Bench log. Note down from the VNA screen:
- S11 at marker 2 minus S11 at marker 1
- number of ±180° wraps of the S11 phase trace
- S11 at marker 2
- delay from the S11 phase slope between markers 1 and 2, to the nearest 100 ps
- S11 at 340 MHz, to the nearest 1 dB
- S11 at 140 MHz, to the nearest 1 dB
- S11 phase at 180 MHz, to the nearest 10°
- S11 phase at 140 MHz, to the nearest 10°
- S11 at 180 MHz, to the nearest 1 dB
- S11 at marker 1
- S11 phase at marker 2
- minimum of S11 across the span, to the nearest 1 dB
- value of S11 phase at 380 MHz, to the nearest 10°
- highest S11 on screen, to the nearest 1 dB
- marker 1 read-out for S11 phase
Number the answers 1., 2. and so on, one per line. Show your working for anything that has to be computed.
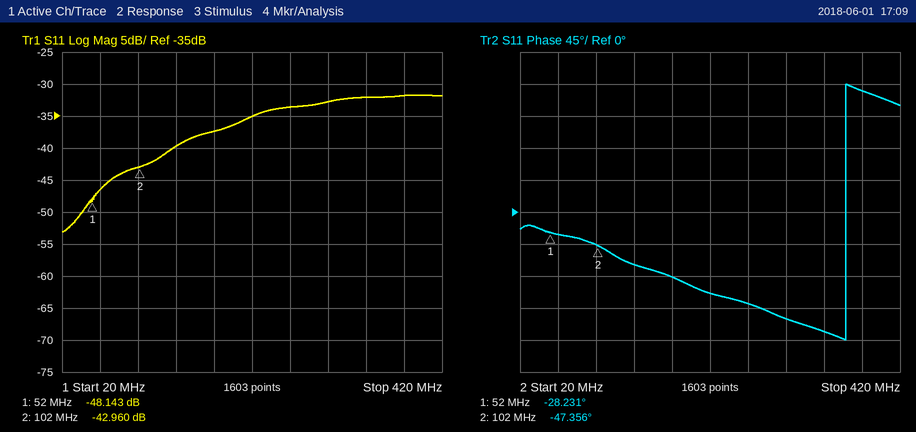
1. -42.96 − (-48.143) = 5.183 dB
2. 1
3. -42.960 dB
4. −(-47.356° − (-28.231°))/(360° × 50 MHz) ≈ 1.1 ns
5. -32 dB
6. -40 dB
7. -90°
8. -70°
9. -37 dB
10. -48.143 dB
11. -47.356°
12. -53 dB
13. 170°
14. -32 dB
15. -28.231°
